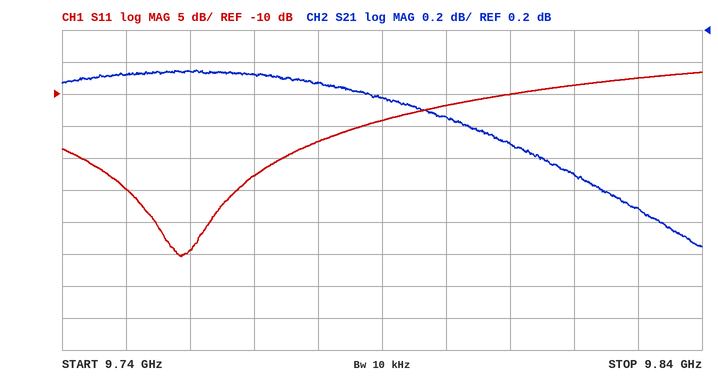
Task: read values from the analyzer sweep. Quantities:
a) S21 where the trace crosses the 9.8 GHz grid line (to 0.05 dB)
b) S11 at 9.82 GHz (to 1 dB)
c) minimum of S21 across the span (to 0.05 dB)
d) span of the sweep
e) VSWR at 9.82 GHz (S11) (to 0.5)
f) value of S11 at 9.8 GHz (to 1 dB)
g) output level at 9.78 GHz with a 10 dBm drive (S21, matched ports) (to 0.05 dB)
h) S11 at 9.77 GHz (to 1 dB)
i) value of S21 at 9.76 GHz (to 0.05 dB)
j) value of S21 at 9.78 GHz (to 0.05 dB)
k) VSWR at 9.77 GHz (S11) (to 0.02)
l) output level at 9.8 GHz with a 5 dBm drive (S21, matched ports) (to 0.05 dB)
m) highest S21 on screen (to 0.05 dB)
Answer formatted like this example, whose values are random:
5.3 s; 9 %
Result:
-0.35 dB; -9 dB; -1.15 dB; 100 MHz; 2.0; -12 dB; 9.85 dBm; -23 dB; -0.05 dB; -0.15 dB; 1.16; 4.65 dBm; -0.05 dB
